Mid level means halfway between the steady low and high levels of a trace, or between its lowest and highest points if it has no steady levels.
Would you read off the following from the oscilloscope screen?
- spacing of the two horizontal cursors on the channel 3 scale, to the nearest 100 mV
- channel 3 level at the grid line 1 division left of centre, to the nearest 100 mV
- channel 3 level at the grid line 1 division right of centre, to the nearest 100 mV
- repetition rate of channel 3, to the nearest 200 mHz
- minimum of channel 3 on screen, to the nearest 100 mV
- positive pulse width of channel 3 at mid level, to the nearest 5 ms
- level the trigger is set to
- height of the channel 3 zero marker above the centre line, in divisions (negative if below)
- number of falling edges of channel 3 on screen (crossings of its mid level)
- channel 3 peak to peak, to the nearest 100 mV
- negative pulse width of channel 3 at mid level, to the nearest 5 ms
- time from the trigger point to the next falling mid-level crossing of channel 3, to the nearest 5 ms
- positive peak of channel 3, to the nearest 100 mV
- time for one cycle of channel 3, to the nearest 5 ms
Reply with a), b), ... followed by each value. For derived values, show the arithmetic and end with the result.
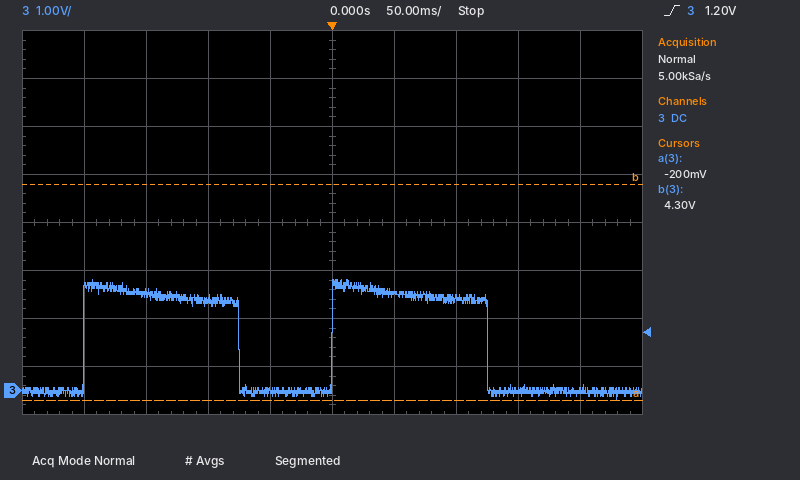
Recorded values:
a) 4.5 V
b) 0.0 V
c) 2.0 V
d) 1 / 200 ms ≈ 5.0 Hz
e) -200 mV
f) 125 ms
g) 1.20 V
h) -3.5 div
i) 2
j) 2.3 V − (-200 mV) = 2.5 V
k) 75 ms
l) 125 ms
m) 2.3 V
n) 200 ms
